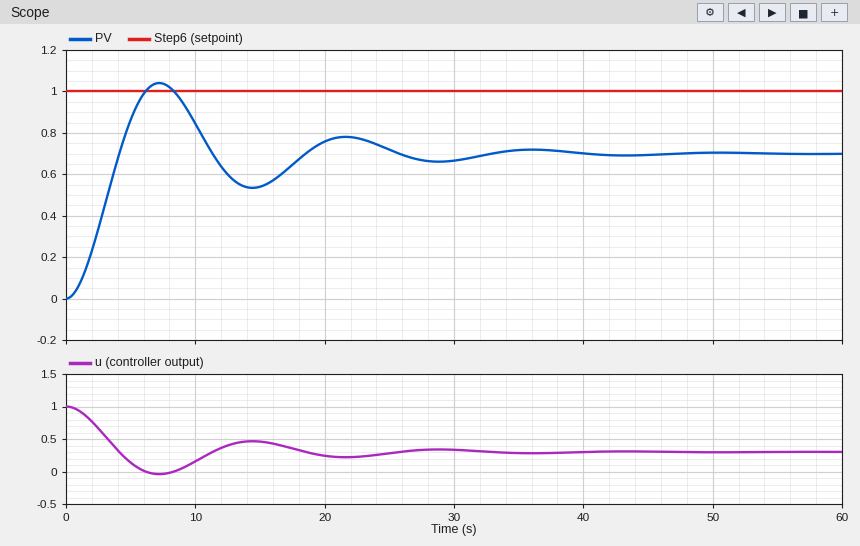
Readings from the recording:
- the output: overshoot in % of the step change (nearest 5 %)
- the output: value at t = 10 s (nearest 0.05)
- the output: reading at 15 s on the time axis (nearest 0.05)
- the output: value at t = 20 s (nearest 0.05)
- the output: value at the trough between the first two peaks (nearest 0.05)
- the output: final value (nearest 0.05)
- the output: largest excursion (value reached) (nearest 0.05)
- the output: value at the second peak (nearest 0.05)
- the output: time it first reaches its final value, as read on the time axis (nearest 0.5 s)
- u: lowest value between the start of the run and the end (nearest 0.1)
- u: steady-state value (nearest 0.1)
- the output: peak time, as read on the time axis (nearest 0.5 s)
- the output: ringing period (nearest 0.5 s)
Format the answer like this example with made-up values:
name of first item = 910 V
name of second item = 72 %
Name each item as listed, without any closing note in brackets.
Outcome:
the output: overshoot in % of the step change = 50 %
the output: value at t = 10 s = 0.85
the output: reading at 15 s on the time axis = 0.55
the output: value at t = 20 s = 0.75
the output: value at the trough between the first two peaks = 0.55
the output: final value = 0.70
the output: largest excursion (value reached) = 1.05
the output: value at the second peak = 0.80
the output: time it first reaches its final value, as read on the time axis = 4.0 s
u: lowest value between the start of the run and the end = 0.0
u: steady-state value = 0.3
the output: peak time, as read on the time axis = 7.0 s
the output: ringing period = 14.5 s
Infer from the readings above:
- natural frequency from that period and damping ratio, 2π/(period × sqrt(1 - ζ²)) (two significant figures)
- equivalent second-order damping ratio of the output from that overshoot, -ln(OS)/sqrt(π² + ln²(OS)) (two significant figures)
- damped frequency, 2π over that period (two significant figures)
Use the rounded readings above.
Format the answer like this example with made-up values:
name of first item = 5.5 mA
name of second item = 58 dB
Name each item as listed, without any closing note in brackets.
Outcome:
natural frequency from that period and damping ratio, 2π/(period × sqrt(1 - ζ²)) = 0.44 rad/s
equivalent second-order damping ratio of the output from that overshoot, -ln(OS)/sqrt(π² + ln²(OS)) = 0.22
damped frequency, 2π over that period = 0.43 rad/s
